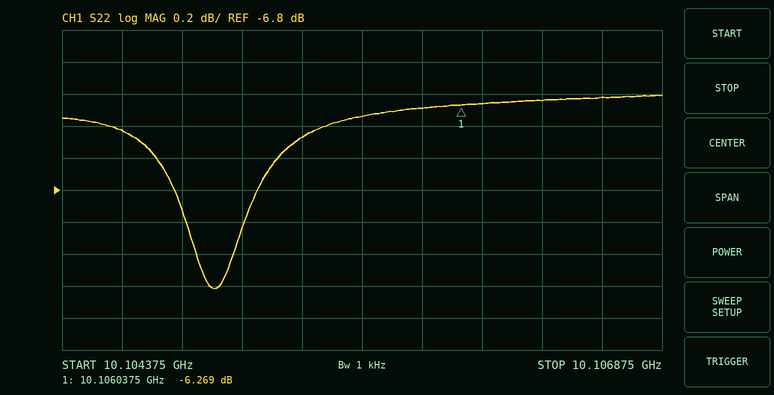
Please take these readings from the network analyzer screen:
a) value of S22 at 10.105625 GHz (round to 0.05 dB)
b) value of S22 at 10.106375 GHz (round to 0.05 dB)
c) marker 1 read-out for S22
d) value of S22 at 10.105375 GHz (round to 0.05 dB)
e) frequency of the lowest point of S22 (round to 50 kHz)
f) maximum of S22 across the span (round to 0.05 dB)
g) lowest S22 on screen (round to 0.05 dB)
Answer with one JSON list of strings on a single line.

["-6.35 dB", "-6.25 dB", "-6.269 dB", "-6.45 dB", "10.10500 GHz", "-6.20 dB", "-7.40 dB"]
